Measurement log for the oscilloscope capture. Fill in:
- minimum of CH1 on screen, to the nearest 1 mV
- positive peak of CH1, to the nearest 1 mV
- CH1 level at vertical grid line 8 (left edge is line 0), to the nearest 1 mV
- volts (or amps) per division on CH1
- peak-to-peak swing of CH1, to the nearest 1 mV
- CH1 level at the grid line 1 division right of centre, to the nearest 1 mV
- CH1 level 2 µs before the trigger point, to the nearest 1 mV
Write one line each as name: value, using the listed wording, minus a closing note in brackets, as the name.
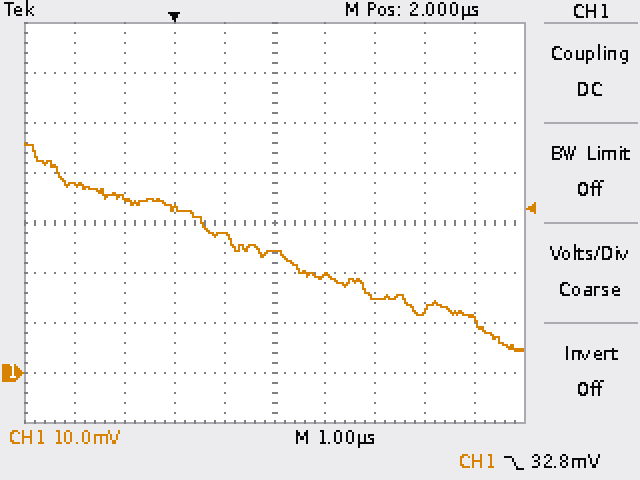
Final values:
minimum of CH1 on screen, to the nearest 1 mV: 4 mV
positive peak of CH1, to the nearest 1 mV: 46 mV
CH1 level at vertical grid line 8 (left edge is line 0), to the nearest 1 mV: 13 mV
volts (or amps) per division on CH1: 10 mV
peak-to-peak swing of CH1, to the nearest 1 mV: 42 mV
CH1 level at the grid line 1 division right of centre, to the nearest 1 mV: 19 mV
CH1 level 2 µs before the trigger point, to the nearest 1 mV: 38 mV
